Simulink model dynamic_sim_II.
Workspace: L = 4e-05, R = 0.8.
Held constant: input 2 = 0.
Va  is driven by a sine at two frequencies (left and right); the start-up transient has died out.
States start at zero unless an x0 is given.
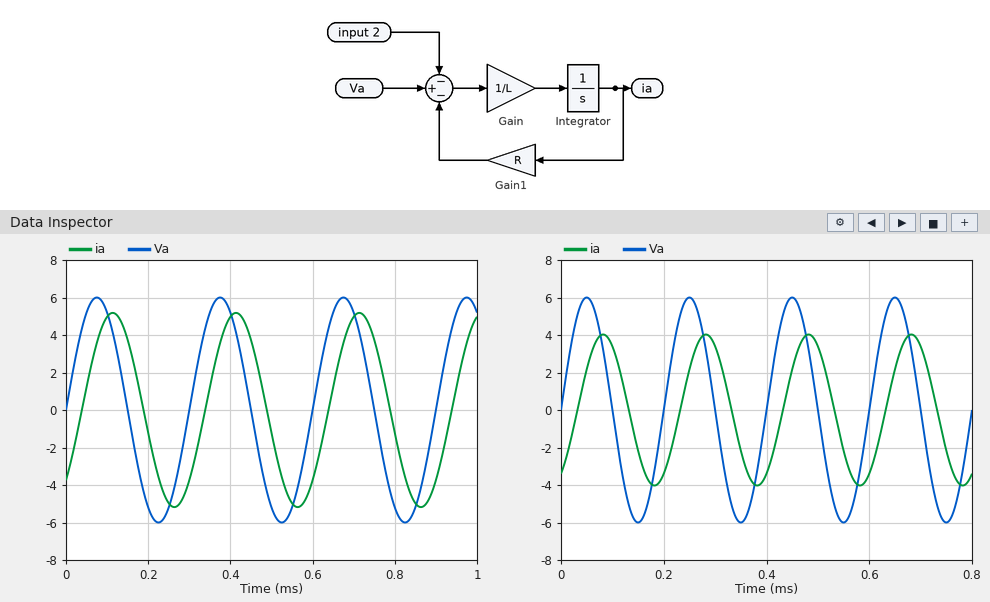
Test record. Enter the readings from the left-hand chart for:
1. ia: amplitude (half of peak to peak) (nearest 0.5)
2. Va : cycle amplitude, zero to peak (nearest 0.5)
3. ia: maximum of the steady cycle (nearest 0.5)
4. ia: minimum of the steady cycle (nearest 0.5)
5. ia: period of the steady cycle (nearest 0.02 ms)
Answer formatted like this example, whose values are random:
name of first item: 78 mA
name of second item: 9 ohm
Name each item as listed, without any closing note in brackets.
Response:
ia: amplitude (half of peak to peak): 5.0
Va : cycle amplitude, zero to peak: 6.0
ia: maximum of the steady cycle: 5.0
ia: minimum of the steady cycle: -5.0
ia: period of the steady cycle: 0.30 ms
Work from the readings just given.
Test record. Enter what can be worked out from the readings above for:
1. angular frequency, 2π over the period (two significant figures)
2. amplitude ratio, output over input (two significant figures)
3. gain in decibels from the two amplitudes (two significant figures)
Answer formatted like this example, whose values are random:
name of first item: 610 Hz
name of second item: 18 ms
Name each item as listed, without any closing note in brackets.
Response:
angular frequency, 2π over the period: 21 rad/ms
amplitude ratio, output over input: 0.83
gain in decibels from the two amplitudes: -1.6 dB
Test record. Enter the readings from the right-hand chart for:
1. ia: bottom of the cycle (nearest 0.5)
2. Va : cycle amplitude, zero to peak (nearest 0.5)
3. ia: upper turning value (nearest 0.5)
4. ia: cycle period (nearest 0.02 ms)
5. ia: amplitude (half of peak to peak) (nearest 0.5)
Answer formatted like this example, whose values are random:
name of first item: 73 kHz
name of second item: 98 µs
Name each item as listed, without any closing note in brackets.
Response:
ia: bottom of the cycle: -4.0
Va : cycle amplitude, zero to peak: 6.0
ia: upper turning value: 4.0
ia: cycle period: 0.20 ms
ia: amplitude (half of peak to peak): 4.0
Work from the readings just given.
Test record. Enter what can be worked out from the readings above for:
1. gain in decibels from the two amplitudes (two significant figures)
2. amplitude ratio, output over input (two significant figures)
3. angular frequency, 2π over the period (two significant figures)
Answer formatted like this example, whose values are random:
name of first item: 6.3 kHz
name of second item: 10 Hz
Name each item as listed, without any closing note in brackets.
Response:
gain in decibels from the two amplitudes: -3.5 dB
amplitude ratio, output over input: 0.67
angular frequency, 2π over the period: 31 rad/ms
